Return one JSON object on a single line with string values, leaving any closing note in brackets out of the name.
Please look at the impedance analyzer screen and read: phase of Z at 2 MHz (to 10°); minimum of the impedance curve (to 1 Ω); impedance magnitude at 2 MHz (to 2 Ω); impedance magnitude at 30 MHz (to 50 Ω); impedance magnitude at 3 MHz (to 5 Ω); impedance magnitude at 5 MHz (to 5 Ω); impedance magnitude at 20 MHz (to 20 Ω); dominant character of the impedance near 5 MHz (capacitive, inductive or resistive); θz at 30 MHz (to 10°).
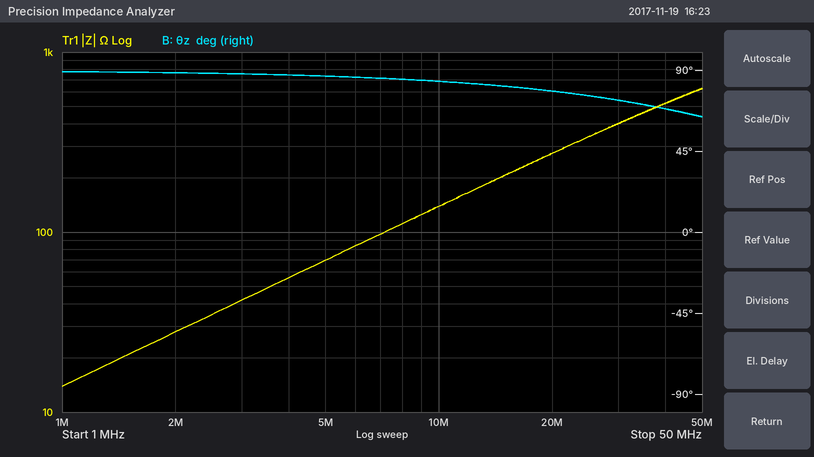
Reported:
{"phase of Z at 2 MHz": "90°", "minimum of the impedance curve": "14 Ω", "impedance magnitude at 2 MHz": "28 Ω", "impedance magnitude at 30 MHz": "400 Ω", "impedance magnitude at 3 MHz": "40 Ω", "impedance magnitude at 5 MHz": "70 Ω", "impedance magnitude at 20 MHz": "280 Ω", "dominant character of the impedance near 5 MHz": "inductive", "θz at 30 MHz": "70°"}
